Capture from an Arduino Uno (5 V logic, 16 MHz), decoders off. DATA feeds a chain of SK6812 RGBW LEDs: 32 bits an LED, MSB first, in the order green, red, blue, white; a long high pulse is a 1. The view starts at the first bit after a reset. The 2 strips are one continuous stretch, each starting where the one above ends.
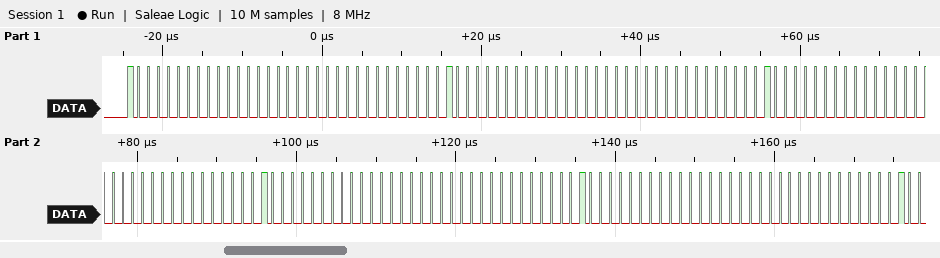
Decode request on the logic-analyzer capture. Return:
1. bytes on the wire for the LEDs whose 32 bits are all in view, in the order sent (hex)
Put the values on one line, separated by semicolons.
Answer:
80 00 00 00 80 00 00 00 80 00 00 00 80 00 00 00 80 00 00 00
